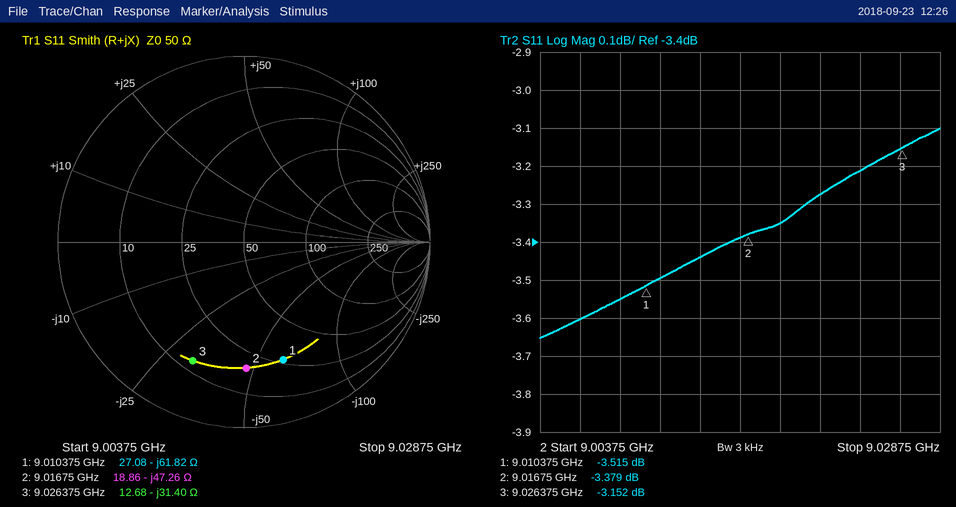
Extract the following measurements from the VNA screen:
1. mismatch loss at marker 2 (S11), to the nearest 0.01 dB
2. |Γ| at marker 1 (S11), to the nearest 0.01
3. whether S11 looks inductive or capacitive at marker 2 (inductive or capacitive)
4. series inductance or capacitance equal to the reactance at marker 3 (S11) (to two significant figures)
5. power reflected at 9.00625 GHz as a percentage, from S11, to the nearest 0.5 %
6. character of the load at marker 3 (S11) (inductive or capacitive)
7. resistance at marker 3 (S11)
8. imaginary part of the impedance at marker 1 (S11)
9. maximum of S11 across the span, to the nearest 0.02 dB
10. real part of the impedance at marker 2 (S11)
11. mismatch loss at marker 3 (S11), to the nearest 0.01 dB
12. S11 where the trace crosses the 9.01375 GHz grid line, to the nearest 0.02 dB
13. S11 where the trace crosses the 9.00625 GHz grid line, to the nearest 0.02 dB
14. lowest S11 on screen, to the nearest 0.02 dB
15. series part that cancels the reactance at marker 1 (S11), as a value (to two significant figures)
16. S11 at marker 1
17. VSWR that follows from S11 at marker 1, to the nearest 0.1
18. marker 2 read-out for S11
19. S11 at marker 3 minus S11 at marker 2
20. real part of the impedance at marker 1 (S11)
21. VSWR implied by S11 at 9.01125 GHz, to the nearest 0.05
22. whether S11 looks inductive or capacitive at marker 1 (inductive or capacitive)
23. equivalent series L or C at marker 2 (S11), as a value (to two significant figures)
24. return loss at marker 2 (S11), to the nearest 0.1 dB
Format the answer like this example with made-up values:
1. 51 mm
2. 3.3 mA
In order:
1. 2.67 dB
2. 0.67
3. capacitive
4. 560 fF
5. 43.5 %
6. capacitive
7. 12.68 Ω
8. -61.82 Ω
9. -3.10 dB
10. 18.86 Ω
11. 2.87 dB
12. -3.44 dB
13. -3.60 dB
14. -3.66 dB
15. 1.1 nH
16. -3.515 dB
17. 5.0
18. -3.379 dB
19. 0.227 dB
20. 27.08 Ω
21. 5.05
22. capacitive
23. 370 fF
24. 3.4 dB
